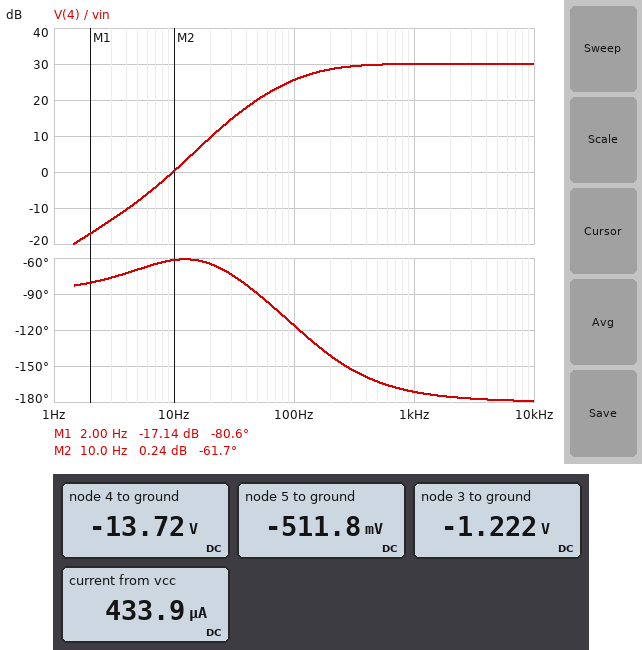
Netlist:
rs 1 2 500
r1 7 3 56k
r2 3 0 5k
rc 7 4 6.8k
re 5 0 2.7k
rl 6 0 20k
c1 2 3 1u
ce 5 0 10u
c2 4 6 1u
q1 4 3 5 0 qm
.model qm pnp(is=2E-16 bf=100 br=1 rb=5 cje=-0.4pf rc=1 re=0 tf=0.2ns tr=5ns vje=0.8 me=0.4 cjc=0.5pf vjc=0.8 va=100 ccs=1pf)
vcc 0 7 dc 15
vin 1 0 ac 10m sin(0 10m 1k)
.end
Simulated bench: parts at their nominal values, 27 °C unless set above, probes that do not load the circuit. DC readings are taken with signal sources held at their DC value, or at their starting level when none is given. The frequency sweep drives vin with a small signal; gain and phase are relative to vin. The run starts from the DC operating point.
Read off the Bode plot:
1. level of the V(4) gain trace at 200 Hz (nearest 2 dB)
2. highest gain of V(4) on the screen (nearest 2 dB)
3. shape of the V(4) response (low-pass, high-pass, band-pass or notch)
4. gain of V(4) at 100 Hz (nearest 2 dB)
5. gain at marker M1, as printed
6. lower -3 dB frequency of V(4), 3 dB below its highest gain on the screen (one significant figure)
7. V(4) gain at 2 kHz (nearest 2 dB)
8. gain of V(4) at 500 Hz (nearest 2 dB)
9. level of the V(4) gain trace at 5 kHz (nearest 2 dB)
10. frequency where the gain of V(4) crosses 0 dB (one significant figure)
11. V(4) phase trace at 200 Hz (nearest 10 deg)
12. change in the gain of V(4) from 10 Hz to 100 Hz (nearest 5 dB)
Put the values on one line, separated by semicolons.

28 dB; 30 dB; high-pass; 26 dB; -17.14 dB; 100 Hz; 30 dB; 30 dB; 30 dB; 10 Hz; -140 deg; 25 dB
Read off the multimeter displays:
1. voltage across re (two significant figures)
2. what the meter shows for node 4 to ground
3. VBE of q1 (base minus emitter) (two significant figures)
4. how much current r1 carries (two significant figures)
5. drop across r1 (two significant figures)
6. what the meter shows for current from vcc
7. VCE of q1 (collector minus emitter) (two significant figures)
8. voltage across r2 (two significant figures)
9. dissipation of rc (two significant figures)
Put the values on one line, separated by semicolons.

510 mV; -13.72 V; -710 mV; 250 µA; 14 V; 433.9 µA; -13 V; 1.2 V; 240 µW
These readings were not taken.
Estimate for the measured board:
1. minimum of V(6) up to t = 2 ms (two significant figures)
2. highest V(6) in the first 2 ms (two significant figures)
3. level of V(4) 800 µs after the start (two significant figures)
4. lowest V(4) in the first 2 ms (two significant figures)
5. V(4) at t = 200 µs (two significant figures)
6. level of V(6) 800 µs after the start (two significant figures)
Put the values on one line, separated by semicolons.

-270 mV; 400 mV; -13 V; -14 V; -14 V; 340 mV
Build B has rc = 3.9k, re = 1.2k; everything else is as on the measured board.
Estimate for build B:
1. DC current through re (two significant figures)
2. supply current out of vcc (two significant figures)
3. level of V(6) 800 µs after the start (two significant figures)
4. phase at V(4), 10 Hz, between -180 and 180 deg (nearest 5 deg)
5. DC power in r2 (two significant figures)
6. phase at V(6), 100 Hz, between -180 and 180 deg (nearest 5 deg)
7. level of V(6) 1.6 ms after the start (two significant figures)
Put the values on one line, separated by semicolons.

400 µA; 650 µA; 390 mV; -80 deg; 290 µW; -100 deg; 340 mV
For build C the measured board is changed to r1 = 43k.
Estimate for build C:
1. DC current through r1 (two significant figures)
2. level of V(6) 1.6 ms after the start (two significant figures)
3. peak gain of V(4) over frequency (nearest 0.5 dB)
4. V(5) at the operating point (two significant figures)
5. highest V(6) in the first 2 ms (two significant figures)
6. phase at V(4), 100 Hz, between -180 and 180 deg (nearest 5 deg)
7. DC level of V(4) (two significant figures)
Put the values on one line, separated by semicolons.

310 µA; 400 mV; 34.0 dB; -830 mV; 610 mV; -105 deg; -13 V
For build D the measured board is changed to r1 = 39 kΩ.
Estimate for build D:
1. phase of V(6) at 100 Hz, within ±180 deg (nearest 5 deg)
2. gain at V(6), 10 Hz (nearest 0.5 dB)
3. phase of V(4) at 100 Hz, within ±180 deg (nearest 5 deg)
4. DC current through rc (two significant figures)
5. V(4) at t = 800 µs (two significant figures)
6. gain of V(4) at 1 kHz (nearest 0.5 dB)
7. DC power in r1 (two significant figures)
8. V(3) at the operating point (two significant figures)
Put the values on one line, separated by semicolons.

-95 deg; -2.0 dB; -100 deg; 350 µA; -12 V; 35.0 dB; 4.5 mW; -1.7 V
